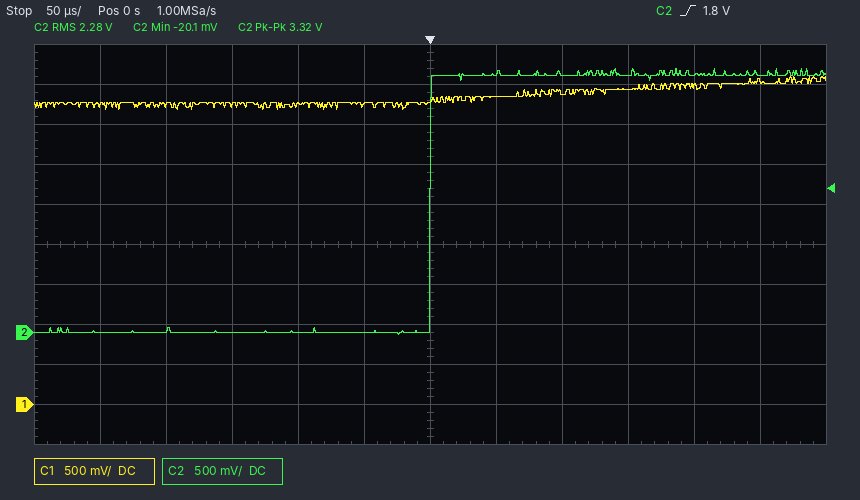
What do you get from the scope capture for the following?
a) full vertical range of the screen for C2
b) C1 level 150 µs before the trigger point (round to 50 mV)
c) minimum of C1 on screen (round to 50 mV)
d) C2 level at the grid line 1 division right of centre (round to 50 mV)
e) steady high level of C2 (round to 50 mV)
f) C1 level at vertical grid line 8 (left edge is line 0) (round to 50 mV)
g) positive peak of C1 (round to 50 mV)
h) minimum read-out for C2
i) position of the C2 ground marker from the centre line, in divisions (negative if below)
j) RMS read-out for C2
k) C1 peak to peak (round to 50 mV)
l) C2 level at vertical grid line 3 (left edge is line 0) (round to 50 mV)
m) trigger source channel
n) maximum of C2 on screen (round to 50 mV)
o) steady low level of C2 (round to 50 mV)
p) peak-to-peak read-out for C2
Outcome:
5 V
3.75 V
3.70 V
3.25 V
3.20 V
3.90 V
4.10 V
-20.1 mV
-2.2 div
2.28 V
400 mV
0 mV
C2
3.30 V
0 mV
3.32 V
